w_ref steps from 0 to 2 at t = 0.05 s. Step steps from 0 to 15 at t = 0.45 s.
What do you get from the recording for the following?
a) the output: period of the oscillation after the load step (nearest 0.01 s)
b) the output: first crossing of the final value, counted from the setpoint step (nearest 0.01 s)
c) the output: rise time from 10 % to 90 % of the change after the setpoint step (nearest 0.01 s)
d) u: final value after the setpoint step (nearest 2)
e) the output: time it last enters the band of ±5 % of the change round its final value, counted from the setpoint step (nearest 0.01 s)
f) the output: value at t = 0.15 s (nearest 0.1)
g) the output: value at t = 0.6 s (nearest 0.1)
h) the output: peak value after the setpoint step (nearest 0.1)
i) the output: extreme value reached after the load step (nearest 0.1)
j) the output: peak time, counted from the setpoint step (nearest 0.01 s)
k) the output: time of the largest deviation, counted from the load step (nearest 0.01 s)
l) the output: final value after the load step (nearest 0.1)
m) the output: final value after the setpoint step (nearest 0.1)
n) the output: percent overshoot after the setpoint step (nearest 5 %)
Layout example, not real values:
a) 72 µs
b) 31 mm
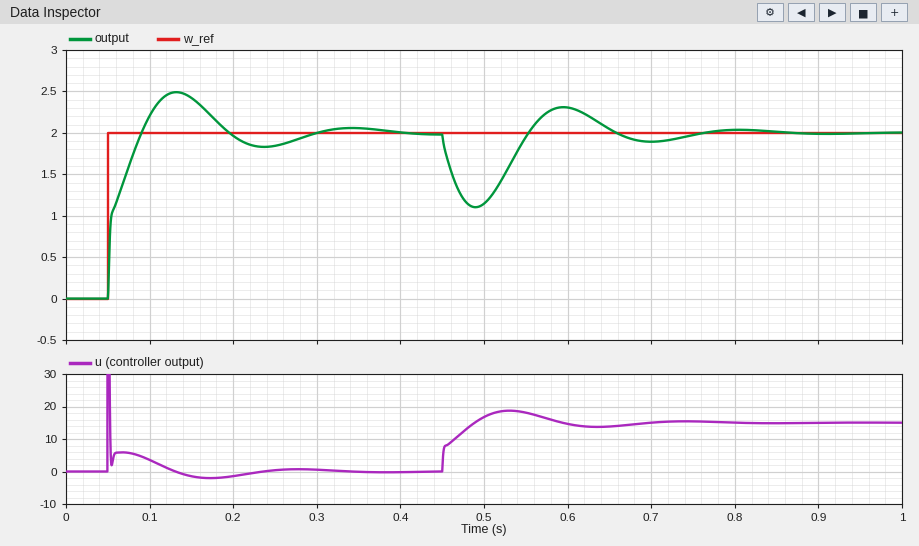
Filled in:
a) 0.21 s
b) 0.04 s
c) 0.03 s
d) 0
e) 0.22 s
f) 2.4
g) 2.3
h) 2.5
i) 1.1
j) 0.08 s
k) 0.04 s
l) 2.0
m) 2.0
n) 25 %
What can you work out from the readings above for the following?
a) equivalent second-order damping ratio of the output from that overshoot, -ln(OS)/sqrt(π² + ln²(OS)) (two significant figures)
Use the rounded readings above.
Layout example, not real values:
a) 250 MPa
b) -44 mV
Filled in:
a) 0.40
